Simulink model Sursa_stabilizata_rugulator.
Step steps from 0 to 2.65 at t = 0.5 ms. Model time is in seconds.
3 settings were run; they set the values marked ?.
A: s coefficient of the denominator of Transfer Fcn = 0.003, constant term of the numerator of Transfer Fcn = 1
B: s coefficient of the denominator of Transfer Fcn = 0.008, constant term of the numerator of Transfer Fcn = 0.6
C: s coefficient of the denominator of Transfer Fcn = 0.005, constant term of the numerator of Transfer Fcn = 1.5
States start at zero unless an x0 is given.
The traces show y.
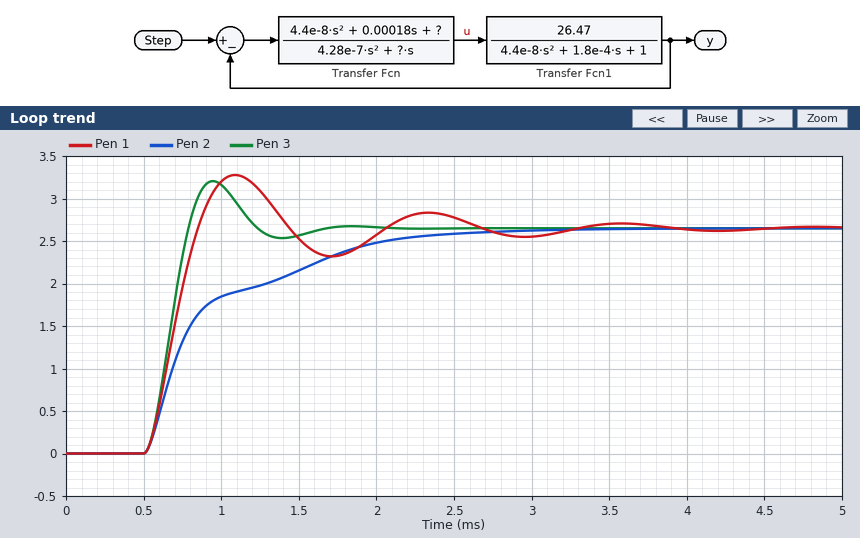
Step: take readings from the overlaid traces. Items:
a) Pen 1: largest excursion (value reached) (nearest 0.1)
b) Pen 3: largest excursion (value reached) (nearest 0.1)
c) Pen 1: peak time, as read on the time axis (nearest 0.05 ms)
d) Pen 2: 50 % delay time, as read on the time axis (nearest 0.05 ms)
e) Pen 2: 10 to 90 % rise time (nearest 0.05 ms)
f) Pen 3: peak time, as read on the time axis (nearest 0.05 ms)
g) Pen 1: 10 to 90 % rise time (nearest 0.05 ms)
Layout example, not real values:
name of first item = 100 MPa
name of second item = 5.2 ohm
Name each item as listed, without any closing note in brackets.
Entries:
Pen 1: largest excursion (value reached) = 3.3
Pen 3: largest excursion (value reached) = 3.2
Pen 1: peak time, as read on the time axis = 1.10 ms
Pen 2: 50 % delay time, as read on the time axis = 0.75 ms
Pen 2: 10 to 90 % rise time = 1.25 ms
Pen 3: peak time, as read on the time axis = 0.95 ms
Pen 1: 10 to 90 % rise time = 0.25 ms
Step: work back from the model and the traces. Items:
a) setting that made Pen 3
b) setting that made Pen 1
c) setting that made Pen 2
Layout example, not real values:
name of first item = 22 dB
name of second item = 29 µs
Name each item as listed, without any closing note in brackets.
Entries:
setting that made Pen 3 = A
setting that made Pen 1 = C
setting that made Pen 2 = B
